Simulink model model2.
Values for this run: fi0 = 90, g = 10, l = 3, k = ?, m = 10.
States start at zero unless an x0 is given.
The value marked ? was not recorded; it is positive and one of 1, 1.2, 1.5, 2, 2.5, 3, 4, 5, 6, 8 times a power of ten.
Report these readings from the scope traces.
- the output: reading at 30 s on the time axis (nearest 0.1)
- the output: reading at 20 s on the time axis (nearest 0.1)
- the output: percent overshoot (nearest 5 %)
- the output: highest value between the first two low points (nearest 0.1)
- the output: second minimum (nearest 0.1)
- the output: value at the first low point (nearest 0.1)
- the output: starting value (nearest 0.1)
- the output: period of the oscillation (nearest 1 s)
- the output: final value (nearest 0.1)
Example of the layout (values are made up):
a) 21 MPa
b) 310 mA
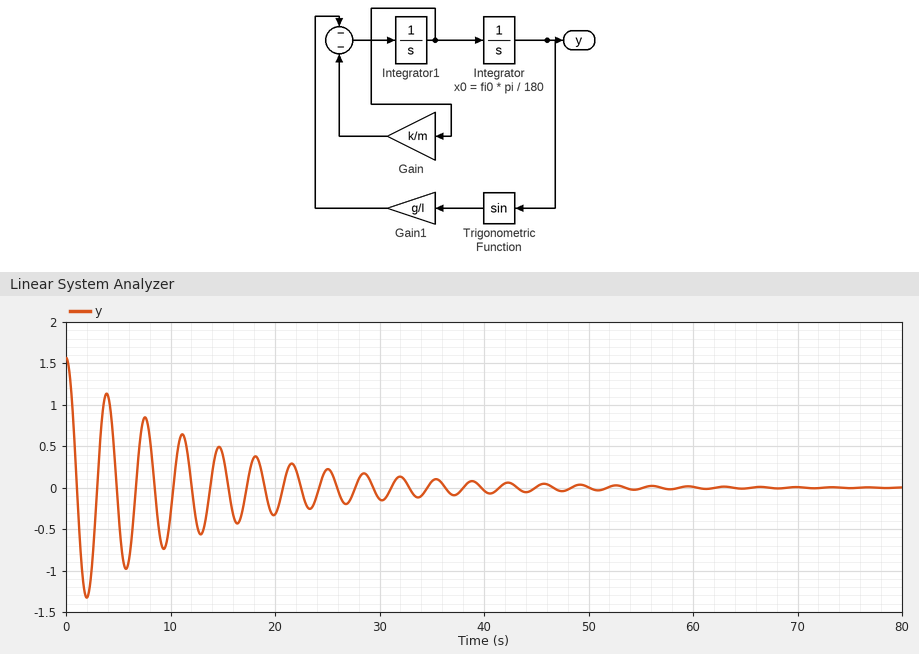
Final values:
a) -0.1
b) -0.3
c) 85 %
d) 1.1
e) -1.0
f) -1.3
g) 1.6
h) 4 s
i) 0.0
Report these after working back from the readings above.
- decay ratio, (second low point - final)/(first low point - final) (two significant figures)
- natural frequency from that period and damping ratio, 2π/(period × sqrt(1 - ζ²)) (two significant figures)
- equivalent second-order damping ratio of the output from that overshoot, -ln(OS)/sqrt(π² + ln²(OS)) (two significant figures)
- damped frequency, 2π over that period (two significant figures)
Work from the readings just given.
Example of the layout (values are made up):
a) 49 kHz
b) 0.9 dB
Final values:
a) 0.77
b) 1.6 rad/s
c) 0.052
d) 1.6 rad/s
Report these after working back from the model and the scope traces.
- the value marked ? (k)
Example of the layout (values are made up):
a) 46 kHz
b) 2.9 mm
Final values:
a) 1.5
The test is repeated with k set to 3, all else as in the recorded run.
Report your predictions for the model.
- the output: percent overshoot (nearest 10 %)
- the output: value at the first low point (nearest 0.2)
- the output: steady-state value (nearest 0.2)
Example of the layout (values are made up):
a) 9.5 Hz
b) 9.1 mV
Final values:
a) 70 %
b) -1.2
c) 0.0
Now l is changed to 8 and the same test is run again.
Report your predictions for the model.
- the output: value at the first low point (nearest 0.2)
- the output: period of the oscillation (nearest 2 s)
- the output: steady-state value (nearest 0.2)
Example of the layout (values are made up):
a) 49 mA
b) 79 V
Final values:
a) -1.2
b) 6 s
c) 0.0
